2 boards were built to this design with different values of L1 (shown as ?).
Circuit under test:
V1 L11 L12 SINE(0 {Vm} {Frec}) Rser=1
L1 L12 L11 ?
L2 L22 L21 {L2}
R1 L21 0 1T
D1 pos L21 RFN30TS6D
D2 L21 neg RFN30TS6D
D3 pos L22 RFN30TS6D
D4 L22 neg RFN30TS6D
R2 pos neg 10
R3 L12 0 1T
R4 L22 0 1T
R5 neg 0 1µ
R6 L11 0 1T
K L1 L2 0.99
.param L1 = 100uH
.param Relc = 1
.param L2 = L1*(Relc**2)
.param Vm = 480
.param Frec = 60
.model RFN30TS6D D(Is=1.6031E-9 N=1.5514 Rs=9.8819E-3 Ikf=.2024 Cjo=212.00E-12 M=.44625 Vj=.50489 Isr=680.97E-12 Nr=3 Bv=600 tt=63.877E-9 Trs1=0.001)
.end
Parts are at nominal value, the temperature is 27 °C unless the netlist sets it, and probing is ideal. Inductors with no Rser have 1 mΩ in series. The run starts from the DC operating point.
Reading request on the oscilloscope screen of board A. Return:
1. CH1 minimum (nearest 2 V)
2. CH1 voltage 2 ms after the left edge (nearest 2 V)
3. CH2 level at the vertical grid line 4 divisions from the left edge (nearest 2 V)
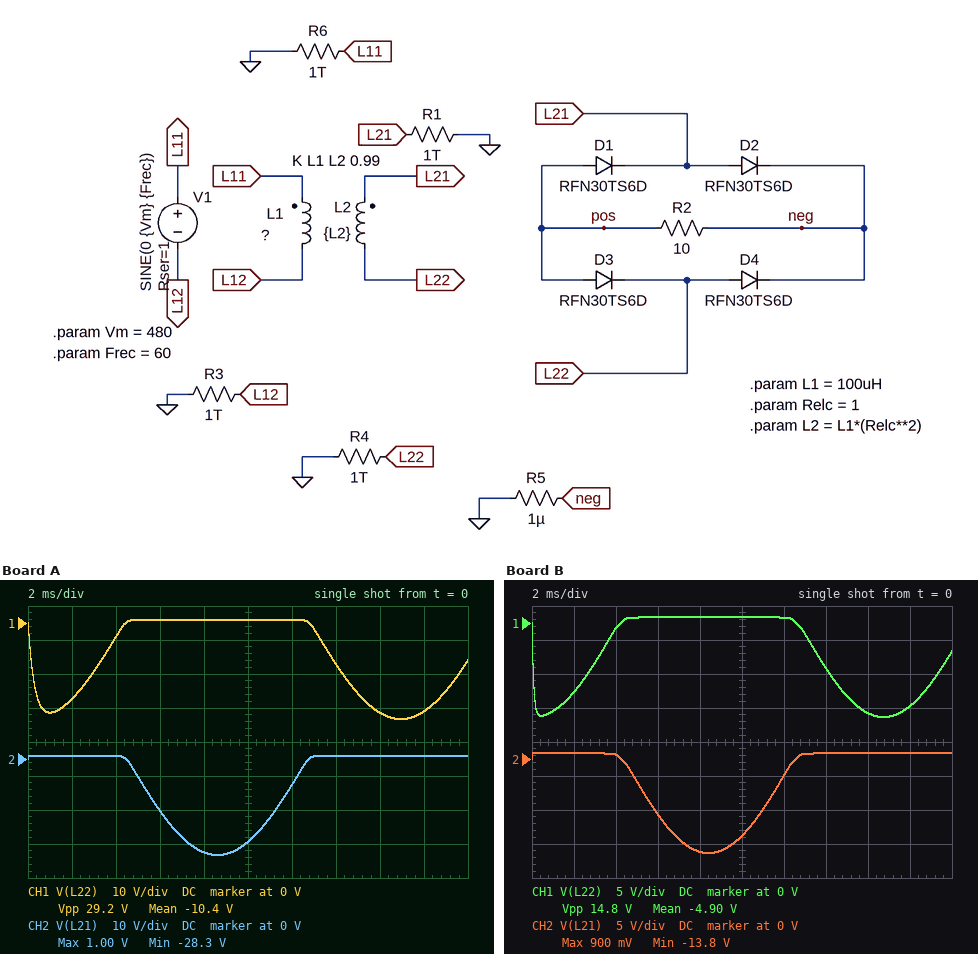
-28 V
-22 V
-28 V
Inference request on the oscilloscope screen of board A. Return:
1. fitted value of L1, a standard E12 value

270 µH
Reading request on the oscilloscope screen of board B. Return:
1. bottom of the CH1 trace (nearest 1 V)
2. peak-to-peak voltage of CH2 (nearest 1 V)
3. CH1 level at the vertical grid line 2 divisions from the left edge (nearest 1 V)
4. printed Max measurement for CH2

-14 V
15 V
-1 V
900 mV
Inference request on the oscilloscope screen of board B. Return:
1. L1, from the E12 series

68 µH
